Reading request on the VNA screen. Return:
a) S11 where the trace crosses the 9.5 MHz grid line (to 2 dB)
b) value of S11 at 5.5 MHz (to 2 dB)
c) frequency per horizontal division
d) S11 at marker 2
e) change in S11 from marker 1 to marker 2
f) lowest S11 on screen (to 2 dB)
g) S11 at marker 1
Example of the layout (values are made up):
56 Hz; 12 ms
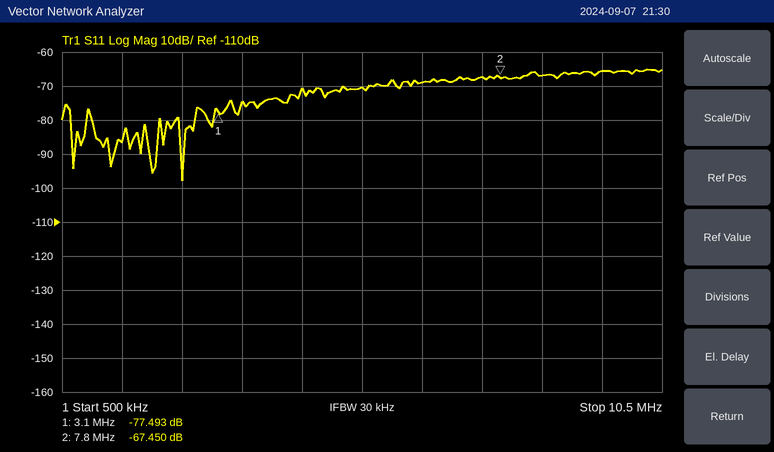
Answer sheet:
-66 dB; -70 dB; 1 MHz; -67.450 dB; 10.043 dB; -98 dB; -77.493 dB
